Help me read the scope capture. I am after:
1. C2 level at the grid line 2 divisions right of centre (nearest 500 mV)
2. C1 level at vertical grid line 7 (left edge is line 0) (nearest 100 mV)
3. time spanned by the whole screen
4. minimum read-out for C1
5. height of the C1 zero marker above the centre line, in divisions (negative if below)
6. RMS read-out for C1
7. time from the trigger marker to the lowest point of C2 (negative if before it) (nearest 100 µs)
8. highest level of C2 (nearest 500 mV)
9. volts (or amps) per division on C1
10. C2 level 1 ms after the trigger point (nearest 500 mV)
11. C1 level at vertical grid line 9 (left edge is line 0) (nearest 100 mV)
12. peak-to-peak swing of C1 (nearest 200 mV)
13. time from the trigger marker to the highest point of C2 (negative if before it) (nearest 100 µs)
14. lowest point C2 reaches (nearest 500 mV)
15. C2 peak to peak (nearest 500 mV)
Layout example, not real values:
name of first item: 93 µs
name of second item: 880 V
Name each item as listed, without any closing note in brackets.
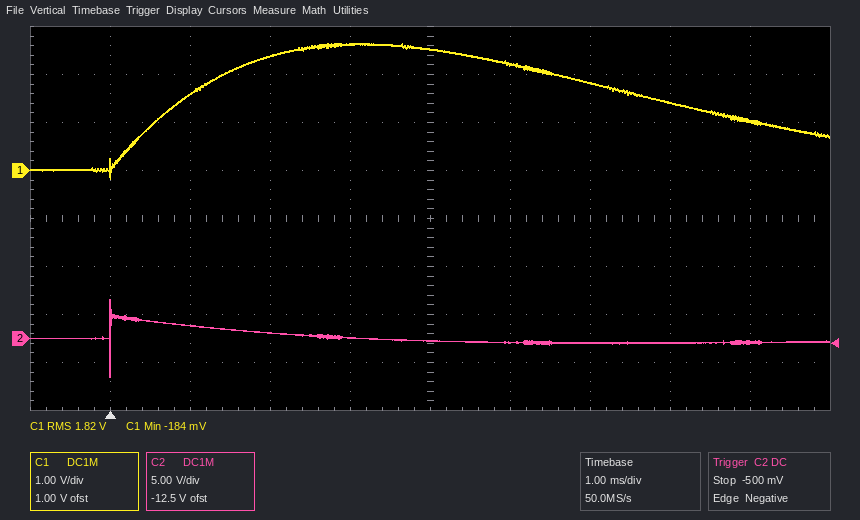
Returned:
C2 level at the grid line 2 divisions right of centre: -500 mV
C1 level at vertical grid line 7 (left edge is line 0): 1.8 V
time spanned by the whole screen: 10 ms
minimum read-out for C1: -184 mV
height of the C1 zero marker above the centre line, in divisions: +1.0 div
RMS read-out for C1: 1.82 V
time from the trigger marker to the lowest point of C2 (negative if before it): 0.0 ms
highest level of C2: 4.0 V
volts (or amps) per division on C1: 1 V
C2 level 1 ms after the trigger point: 1.5 V
C1 level at vertical grid line 9 (left edge is line 0): 1.0 V
peak-to-peak swing of C1: 2.8 V
time from the trigger marker to the highest point of C2 (negative if before it): 0.0 ms
lowest point C2 reaches: -4.0 V
C2 peak to peak: 8.0 V
